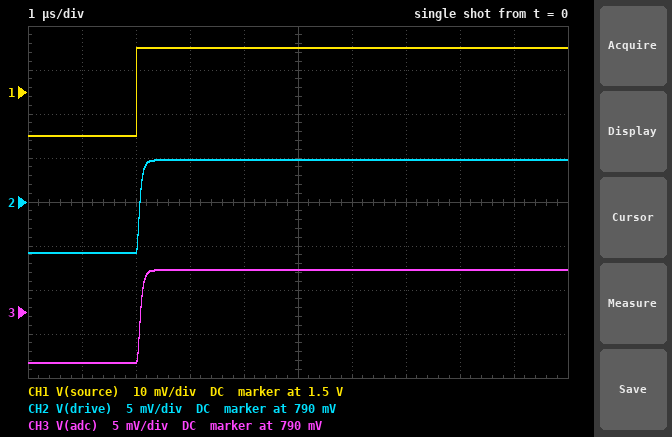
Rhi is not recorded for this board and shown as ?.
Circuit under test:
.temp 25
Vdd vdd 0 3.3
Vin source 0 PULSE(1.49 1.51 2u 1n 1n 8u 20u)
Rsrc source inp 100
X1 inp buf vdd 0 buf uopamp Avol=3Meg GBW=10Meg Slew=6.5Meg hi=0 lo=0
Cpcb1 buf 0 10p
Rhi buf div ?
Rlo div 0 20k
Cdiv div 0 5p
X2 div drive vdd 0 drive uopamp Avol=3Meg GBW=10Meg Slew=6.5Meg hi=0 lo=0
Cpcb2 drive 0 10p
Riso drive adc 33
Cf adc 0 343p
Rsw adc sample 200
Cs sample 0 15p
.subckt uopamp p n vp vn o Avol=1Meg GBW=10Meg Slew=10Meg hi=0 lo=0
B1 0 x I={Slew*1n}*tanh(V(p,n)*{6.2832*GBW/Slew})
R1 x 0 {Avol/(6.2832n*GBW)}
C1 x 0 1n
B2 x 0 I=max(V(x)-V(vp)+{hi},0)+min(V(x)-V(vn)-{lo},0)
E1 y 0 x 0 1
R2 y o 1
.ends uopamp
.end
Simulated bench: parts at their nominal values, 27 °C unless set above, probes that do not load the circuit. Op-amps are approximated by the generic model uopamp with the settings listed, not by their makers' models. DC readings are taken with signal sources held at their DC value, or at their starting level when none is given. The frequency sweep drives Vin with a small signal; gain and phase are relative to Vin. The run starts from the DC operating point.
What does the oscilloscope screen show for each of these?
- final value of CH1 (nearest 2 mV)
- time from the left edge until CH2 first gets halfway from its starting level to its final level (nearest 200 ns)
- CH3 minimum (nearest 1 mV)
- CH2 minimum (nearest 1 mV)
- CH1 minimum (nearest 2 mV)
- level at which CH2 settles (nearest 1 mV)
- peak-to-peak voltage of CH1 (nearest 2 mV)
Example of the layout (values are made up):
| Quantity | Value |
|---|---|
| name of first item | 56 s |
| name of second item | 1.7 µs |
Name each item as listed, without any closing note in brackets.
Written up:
| Quantity | Value |
|---|---|
| final value of CH1 | 1.510 V |
| time from the left edge until CH2 first gets halfway from its starting level to its final level | 2.0 µs |
| CH3 minimum | 784 mV |
| CH2 minimum | 784 mV |
| CH1 minimum | 1.490 V |
| level at which CH2 settles | 795 mV |
| peak-to-peak voltage of CH1 | 20 mV |
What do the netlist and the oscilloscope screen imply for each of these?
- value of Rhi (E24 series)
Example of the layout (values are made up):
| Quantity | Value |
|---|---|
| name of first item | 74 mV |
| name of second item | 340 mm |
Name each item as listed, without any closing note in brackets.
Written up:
| Quantity | Value |
|---|---|
| value of Rhi | 18 kΩ |
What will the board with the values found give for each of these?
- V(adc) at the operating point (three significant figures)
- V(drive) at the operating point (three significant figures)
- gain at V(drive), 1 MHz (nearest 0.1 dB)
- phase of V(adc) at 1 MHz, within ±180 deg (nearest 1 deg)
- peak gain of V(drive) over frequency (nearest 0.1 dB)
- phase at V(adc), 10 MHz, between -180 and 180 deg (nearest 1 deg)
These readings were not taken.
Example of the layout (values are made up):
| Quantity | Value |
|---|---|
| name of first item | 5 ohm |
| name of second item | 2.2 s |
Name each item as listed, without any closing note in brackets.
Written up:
| Quantity | Value |
|---|---|
| V(adc) at the operating point | 784 mV |
| V(drive) at the operating point | 784 mV |
| gain at V(drive), 1 MHz | -6.0 dB |
| phase of V(adc) at 1 MHz, within ±180 deg | -32 deg |
| peak gain of V(drive) over frequency | -5.6 dB |
| phase at V(adc), 10 MHz, between -180 and 180 deg | 161 deg |
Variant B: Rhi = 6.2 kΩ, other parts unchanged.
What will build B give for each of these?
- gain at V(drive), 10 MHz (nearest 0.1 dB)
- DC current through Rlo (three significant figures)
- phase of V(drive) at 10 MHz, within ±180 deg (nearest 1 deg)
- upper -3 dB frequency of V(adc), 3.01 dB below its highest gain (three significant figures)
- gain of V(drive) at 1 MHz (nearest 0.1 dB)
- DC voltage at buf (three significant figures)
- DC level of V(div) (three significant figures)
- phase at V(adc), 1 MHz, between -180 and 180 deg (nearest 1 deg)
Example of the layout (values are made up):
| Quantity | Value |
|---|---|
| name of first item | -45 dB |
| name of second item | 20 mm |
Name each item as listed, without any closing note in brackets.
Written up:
| Quantity | Value |
|---|---|
| gain at V(drive), 10 MHz | -13.4 dB |
| DC current through Rlo | 56.9 µA |
| phase of V(drive) at 10 MHz, within ±180 deg | -147 deg |
| upper -3 dB frequency of V(adc), 3.01 dB below its highest gain | 4.04 MHz |
| gain of V(drive) at 1 MHz | -2.5 dB |
| DC voltage at buf | 1.49 V |
| DC level of V(div) | 1.14 V |
| phase at V(adc), 1 MHz, between -180 and 180 deg | -24 deg |
